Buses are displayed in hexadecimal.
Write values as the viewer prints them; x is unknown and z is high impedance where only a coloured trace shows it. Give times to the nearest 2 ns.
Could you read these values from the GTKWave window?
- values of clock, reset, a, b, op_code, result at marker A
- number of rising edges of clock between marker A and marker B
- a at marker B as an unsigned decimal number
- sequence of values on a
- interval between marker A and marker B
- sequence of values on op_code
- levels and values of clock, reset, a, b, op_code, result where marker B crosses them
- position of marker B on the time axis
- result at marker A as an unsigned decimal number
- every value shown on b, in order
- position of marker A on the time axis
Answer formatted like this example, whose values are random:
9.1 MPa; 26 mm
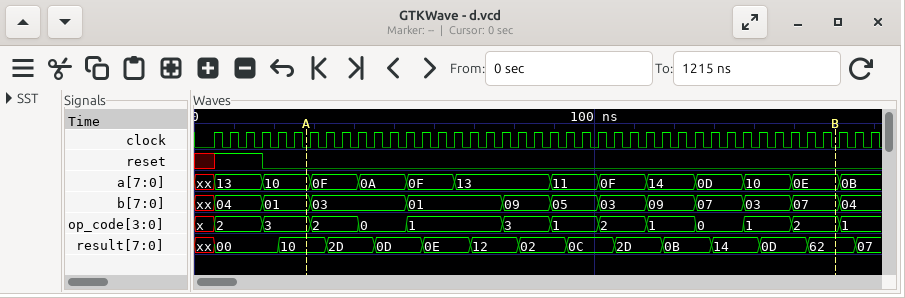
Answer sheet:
clock=0, reset=0, a=10, b=01, op_code=3, result=10; 33; 14; xx, 13, 10, 0F, 0A, 0F, 13, 11, 0F, 14, 0D, 10, 0E, 0B; 132 ns; x, 2, 3, 2, 0, 1, 3, 1, 2, 1, 0, 1, 2, 1; clock=0, reset=0, a=0E, b=07, op_code=2, result=62; 160 ns; 16; xx, 04, 01, 03, 01, 09, 05, 03, 09, 07, 03, 07, 04; 28 ns
